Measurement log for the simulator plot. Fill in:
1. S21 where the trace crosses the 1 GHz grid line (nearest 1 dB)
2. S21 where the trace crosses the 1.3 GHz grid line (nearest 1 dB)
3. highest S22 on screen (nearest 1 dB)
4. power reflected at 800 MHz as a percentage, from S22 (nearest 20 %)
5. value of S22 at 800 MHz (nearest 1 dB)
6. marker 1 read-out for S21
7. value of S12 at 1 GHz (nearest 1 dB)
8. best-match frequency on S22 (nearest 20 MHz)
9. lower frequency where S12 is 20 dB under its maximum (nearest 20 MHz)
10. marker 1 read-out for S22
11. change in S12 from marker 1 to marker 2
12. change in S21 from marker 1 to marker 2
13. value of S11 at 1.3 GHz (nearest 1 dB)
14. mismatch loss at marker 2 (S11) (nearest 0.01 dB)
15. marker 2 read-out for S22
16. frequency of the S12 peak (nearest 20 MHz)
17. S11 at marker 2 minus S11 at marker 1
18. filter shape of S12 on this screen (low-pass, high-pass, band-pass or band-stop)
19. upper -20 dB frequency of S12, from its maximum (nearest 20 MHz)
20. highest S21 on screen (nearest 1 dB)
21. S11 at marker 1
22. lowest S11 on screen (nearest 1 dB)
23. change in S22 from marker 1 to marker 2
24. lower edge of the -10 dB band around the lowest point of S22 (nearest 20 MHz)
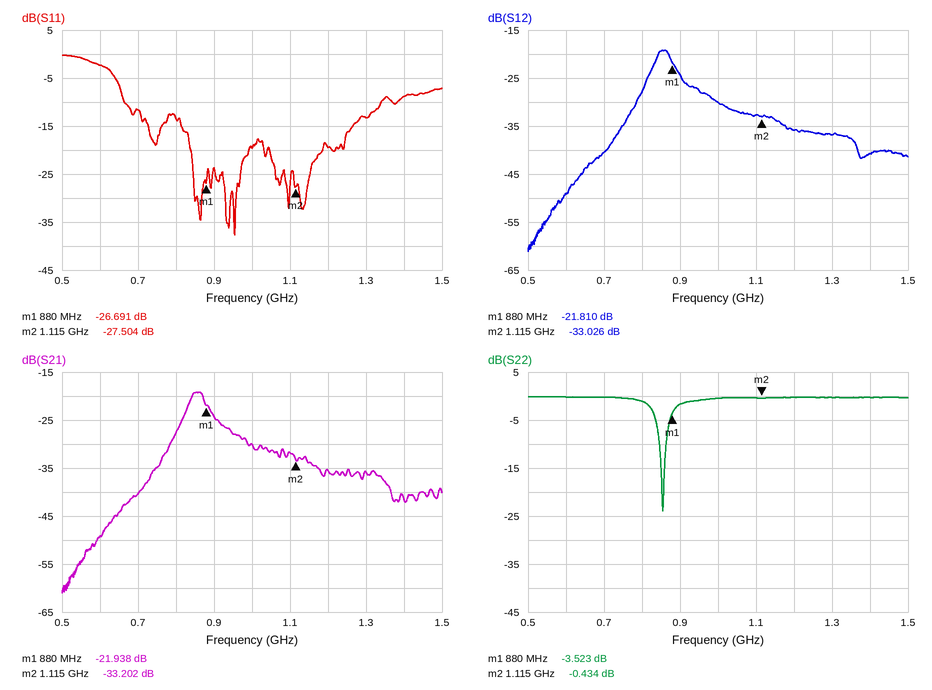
-30 dB
-36 dB
0 dB
80 %
-1 dB
-21.938 dB
-30 dB
860 MHz
720 MHz
-3.523 dB
-11.216 dB
-11.264 dB
-13 dB
0.01 dB
-0.434 dB
860 MHz
-0.813 dB
band-pass
1.36 GHz
-19 dB
-26.691 dB
-38 dB
3.089 dB
840 MHz
